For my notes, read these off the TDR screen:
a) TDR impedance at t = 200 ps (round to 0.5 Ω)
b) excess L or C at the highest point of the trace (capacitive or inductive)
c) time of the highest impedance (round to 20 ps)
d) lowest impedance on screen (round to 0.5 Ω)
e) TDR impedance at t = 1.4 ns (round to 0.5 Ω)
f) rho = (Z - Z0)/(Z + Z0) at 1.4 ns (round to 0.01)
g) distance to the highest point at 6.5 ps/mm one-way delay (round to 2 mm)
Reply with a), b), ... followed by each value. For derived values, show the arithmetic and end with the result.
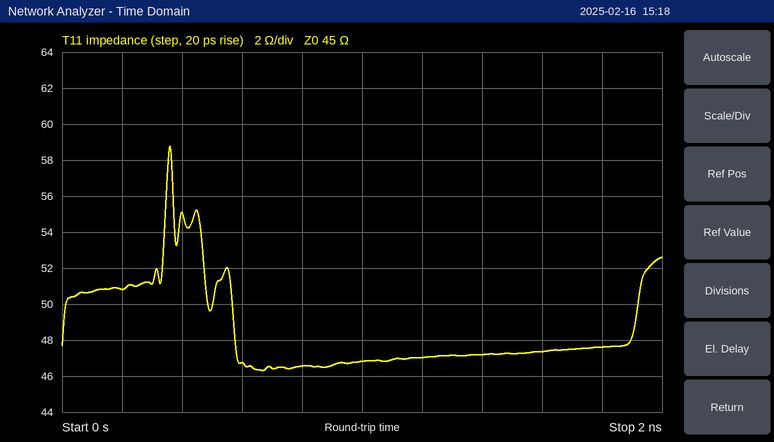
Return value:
a) 51.0 Ω
b) inductive
c) 360 ps
d) 46.5 Ω
e) 47.0 Ω
f) (47 − 45)/(47 + 45) ≈ +0.02
g) 360 ps / 2 / 6.5 ps/mm ≈ 28 mm
